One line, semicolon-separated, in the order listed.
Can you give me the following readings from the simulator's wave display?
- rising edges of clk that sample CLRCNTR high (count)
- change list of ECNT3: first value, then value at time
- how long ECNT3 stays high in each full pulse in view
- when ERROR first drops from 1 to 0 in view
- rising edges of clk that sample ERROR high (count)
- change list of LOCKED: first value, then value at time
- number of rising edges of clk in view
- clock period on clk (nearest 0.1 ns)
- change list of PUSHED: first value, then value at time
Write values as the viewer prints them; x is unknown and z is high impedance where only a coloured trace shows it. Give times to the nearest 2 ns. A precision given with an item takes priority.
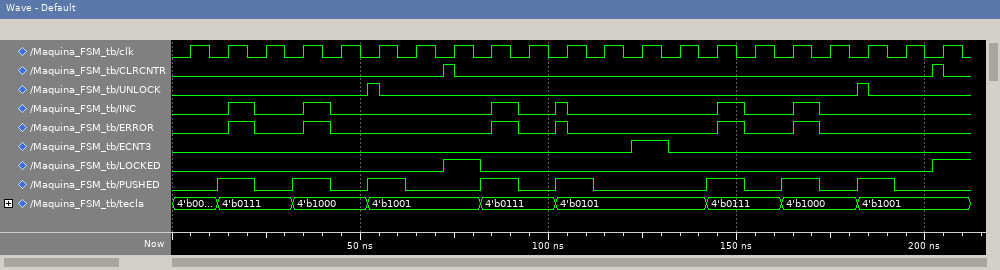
2; 0, 1 at 122 ns, 0 at 132 ns; 10 ns; 22 ns; 1; 0, 1 at 72 ns, 0 at 82 ns, 1 at 202 ns; 21; 10 ns; 0, 1 at 12 ns, 0 at 22 ns, 1 at 32 ns, 0 at 42 ns, 1 at 52 ns, 0 at 62 ns, 1 at 82 ns, 0 at 92 ns, 1 at 102 ns, 0 at 112 ns, 1 at 142 ns, 0 at 152 ns, 1 at 162 ns, 0 at 172 ns, 1 at 182 ns, 0 at 192 ns
